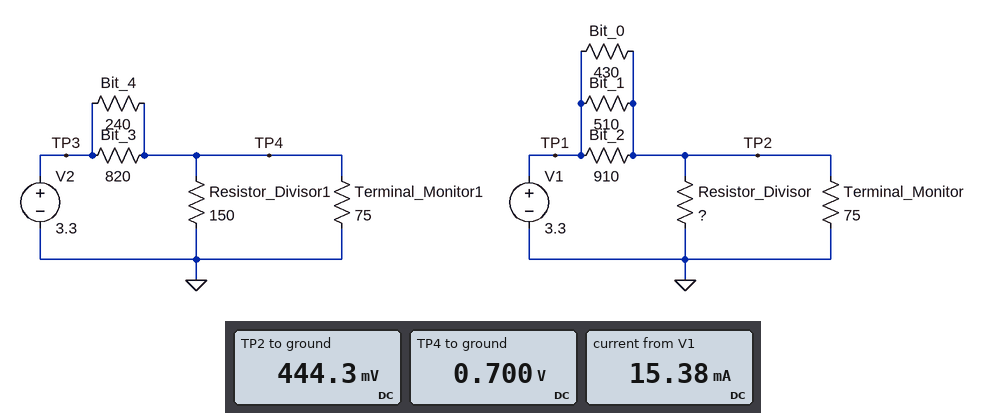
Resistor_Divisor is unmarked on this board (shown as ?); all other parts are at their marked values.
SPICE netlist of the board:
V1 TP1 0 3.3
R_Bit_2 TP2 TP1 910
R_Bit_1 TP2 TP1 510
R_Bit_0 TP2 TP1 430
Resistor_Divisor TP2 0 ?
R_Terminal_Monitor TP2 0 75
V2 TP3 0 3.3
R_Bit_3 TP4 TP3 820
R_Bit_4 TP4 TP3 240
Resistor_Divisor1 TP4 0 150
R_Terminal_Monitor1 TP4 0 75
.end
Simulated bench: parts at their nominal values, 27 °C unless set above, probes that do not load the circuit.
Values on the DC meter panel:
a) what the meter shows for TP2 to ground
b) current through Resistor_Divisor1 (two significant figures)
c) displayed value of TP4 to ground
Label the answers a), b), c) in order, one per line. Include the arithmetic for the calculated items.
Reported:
a) 444.3 mV
b) (700 mV) / 150 Ω = 4.7 mA
c) 0.700 V
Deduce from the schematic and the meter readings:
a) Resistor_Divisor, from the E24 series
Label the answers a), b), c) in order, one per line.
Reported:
a) 47 Ω
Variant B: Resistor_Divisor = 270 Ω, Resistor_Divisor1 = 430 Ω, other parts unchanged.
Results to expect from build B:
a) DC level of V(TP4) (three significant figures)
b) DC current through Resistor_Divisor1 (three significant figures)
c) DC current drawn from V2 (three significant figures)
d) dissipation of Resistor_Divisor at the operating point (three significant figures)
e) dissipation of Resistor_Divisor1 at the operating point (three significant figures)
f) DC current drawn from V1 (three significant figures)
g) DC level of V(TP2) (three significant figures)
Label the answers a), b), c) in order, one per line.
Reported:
a) 845 mV
b) 1.96 mA
c) 13.2 mA
d) 2.33 mW
e) 1.66 mW
f) 13.5 mA
g) 793 mV
